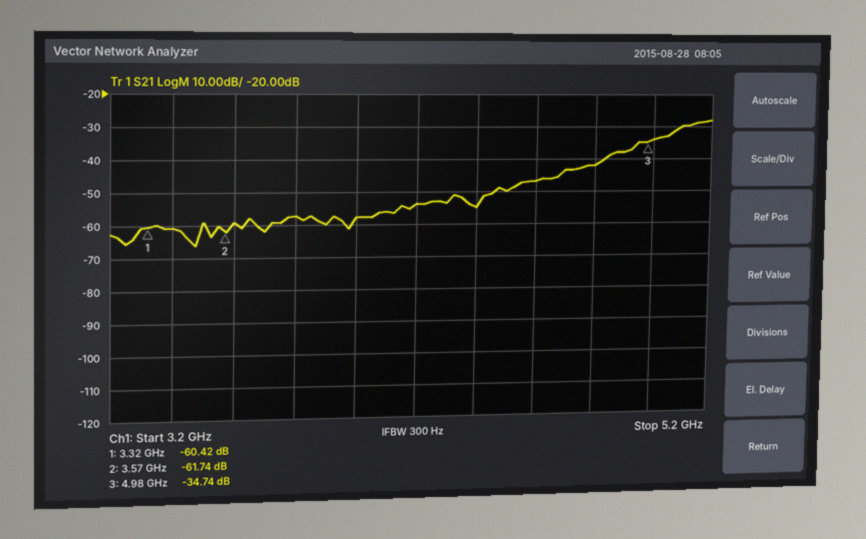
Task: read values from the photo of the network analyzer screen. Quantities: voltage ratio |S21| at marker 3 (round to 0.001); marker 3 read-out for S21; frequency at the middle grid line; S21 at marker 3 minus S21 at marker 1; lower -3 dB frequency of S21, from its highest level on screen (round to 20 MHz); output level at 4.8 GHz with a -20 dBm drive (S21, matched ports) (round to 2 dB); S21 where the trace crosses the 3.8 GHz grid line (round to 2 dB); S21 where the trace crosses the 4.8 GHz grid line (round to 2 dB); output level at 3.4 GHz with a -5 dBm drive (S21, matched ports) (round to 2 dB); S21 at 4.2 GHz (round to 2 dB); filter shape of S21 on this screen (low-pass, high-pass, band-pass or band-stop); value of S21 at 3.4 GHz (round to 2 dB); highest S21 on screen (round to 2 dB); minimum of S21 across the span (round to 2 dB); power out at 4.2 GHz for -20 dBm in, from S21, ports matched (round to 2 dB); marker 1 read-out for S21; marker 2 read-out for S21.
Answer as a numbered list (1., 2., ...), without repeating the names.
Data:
1. 0.018
2. -34.74 dB
3. 4.2 GHz
4. 25.68 dB
5. 5.08 GHz
6. -62 dBm
7. -58 dB
8. -42 dB
9. -66 dBm
10. -54 dB
11. high-pass
12. -60 dB
13. -28 dB
14. -66 dB
15. -74 dBm
16. -60.42 dB
17. -61.74 dB
